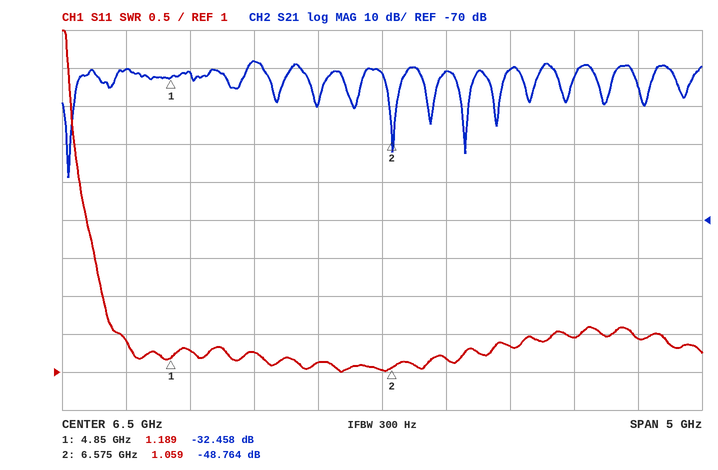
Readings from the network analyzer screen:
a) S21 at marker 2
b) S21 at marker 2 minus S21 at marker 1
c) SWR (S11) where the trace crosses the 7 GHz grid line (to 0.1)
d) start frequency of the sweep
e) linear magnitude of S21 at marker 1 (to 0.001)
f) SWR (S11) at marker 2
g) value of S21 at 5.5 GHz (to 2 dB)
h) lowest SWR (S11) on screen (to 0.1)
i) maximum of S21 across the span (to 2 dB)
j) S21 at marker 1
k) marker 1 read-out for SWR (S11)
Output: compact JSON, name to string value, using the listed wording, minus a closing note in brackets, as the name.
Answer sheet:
{"S21 at marker 2": "-48.764 dB", "S21 at marker 2 minus S21 at marker 1": "-16.306 dB", "SWR (S11) where the trace crosses the 7 GHz grid line": "1.2", "start frequency of the sweep": "4 GHz", "linear magnitude of S21 at marker 1": "0.024", "SWR (S11) at marker 2": "1.059", "value of S21 at 5.5 GHz": "-28 dB", "lowest SWR (S11) on screen": "1.0", "maximum of S21 across the span": "-28 dB", "S21 at marker 1": "-32.458 dB", "marker 1 read-out for SWR": "1.189"}
